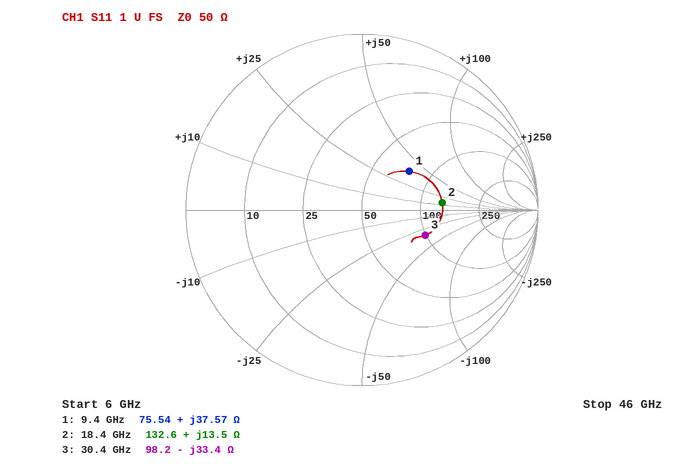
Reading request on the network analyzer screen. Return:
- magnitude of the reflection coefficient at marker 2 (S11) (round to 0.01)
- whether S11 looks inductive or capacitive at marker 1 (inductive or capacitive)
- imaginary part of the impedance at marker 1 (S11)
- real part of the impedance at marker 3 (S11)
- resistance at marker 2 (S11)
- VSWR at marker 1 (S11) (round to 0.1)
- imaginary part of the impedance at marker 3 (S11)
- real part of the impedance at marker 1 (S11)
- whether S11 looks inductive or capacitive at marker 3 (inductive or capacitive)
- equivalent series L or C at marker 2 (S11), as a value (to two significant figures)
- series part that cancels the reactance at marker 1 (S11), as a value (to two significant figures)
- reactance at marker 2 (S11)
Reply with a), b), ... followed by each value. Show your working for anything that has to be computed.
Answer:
a) 0.46
b) inductive
c) +37.57 Ω
d) 98.2 Ω
e) 132.6 Ω
f) 2.1
g) -33.4 Ω
h) 75.54 Ω
i) capacitive
j) L = 13.5 Ω/(2π × 18.4 GHz) ≈ 117 pH, so 120 pH to two significant figures
k) C = 1/(2π × 9.4 GHz × 37.57 Ω) ≈ 451 fF, so 450 fF to two significant figures
l) +13.5 Ω
